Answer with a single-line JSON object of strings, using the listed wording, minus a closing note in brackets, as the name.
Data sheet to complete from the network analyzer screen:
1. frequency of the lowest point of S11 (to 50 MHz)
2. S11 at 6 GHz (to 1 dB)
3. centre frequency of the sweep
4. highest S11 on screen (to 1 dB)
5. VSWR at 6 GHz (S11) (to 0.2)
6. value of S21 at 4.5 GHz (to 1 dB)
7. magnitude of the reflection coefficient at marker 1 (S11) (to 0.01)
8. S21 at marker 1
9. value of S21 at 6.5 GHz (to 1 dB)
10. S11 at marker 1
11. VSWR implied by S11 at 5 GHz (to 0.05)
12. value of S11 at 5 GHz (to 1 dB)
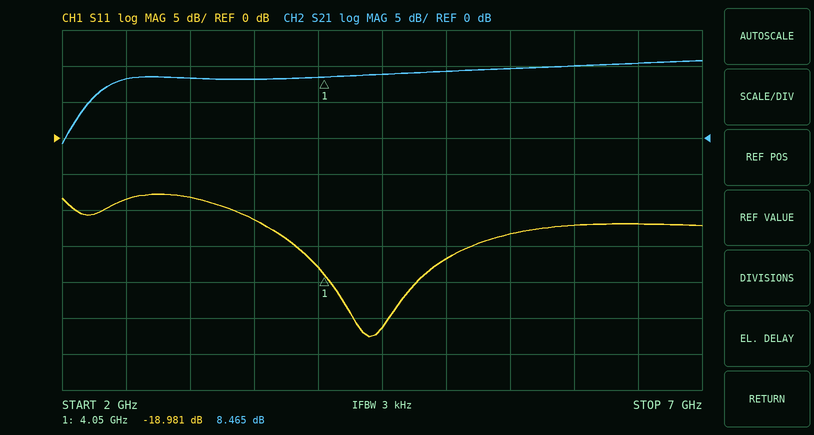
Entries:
{"frequency of the lowest point of S11": "4.40 GHz", "S11 at 6 GHz": "-12 dB", "centre frequency of the sweep": "4.5 GHz", "highest S11 on screen": "-8 dB", "VSWR at 6 GHz (S11)": "1.6", "value of S21 at 4.5 GHz": "9 dB", "magnitude of the reflection coefficient at marker 1 (S11)": "0.11", "S21 at marker 1": "8.465 dB", "value of S21 at 6.5 GHz": "10 dB", "S11 at marker 1": "-18.981 dB", "VSWR implied by S11 at 5 GHz": "1.35", "value of S11 at 5 GHz": "-17 dB"}
